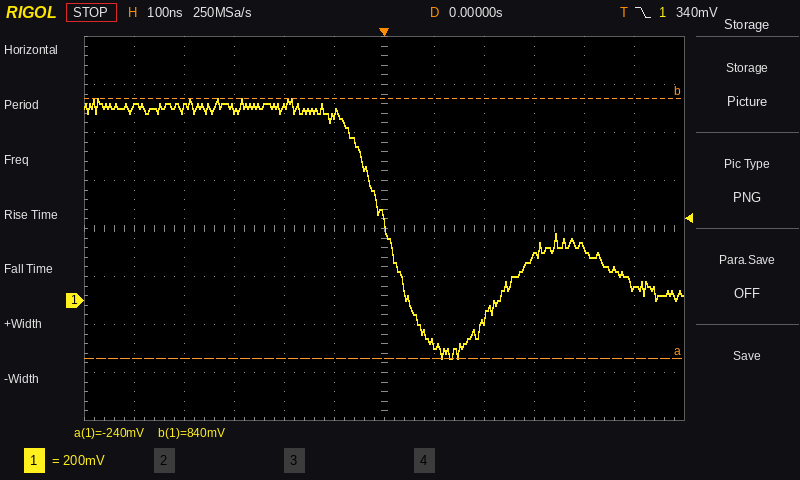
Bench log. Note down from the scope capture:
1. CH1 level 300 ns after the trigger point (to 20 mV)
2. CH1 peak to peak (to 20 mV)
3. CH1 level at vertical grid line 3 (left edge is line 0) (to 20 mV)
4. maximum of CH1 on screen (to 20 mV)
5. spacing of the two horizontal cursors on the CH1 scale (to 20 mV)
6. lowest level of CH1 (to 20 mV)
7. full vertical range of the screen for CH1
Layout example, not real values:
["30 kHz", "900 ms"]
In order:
["180 mV", "1.08 V", "800 mV", "840 mV", "1.08 V", "-240 mV", "1.6 V"]
